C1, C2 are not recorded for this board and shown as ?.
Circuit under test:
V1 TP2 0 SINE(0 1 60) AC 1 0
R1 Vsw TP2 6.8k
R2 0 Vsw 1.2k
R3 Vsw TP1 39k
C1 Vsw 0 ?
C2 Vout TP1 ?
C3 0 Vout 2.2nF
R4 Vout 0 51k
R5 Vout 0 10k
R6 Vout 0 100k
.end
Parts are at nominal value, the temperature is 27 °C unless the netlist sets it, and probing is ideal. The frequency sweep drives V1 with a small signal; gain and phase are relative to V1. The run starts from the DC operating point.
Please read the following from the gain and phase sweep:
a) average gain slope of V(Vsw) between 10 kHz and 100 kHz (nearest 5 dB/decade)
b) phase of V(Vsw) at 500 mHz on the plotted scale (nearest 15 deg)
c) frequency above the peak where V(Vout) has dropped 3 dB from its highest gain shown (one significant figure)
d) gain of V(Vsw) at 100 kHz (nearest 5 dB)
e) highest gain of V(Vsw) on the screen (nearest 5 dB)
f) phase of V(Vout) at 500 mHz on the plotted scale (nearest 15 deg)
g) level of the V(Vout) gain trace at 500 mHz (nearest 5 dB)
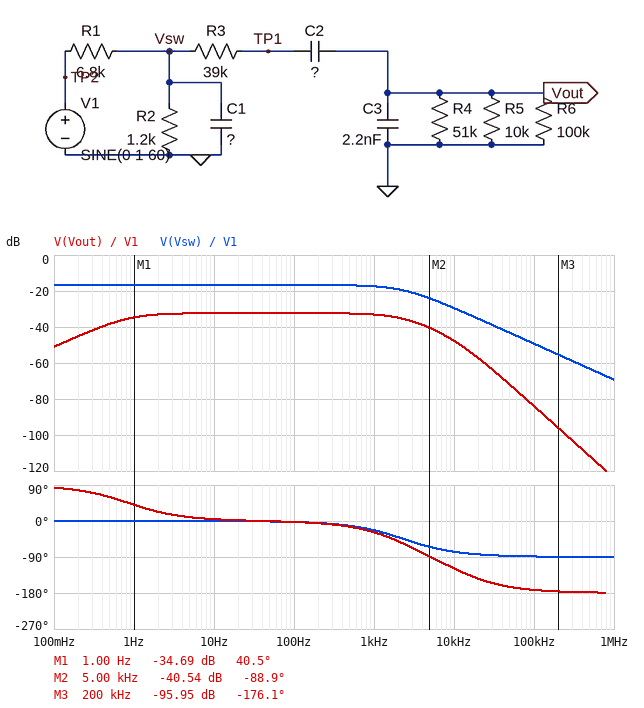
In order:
-20 dB/decade
0 deg
2 kHz
-50 dB
-15 dB
60 deg
-40 dB
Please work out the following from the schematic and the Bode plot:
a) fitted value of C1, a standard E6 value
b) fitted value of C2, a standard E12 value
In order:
68 nF
3.9 µF
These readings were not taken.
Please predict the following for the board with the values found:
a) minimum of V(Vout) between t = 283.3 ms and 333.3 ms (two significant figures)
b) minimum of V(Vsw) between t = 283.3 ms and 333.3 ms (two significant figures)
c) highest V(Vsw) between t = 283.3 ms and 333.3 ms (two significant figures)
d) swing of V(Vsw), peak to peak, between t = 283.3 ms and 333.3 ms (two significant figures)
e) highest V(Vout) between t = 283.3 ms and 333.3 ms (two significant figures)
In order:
-24 mV
-150 mV
150 mV
290 mV
24 mV
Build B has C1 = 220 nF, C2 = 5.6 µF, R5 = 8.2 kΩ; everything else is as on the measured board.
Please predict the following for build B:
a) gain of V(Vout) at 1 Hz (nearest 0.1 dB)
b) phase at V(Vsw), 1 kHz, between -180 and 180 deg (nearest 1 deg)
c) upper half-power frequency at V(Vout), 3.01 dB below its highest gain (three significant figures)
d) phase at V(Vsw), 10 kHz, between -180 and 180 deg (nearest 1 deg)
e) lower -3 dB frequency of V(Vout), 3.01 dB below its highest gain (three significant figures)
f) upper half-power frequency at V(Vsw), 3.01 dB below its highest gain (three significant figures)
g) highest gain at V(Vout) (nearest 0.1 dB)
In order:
-34.8 dB
-54 deg
724 Hz
-86 deg
609 mHz
693 Hz
-33.5 dB
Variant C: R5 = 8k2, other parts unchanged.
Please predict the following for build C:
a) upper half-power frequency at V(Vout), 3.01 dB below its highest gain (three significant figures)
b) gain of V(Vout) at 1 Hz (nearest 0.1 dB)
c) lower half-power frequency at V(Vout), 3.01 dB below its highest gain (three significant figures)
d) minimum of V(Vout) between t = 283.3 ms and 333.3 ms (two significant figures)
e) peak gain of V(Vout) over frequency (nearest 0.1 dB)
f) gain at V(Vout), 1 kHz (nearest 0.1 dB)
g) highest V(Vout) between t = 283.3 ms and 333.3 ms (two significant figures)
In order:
2.27 kHz
-35.9 dB
875 mHz
-21 mV
-33.5 dB
-34.2 dB
21 mV
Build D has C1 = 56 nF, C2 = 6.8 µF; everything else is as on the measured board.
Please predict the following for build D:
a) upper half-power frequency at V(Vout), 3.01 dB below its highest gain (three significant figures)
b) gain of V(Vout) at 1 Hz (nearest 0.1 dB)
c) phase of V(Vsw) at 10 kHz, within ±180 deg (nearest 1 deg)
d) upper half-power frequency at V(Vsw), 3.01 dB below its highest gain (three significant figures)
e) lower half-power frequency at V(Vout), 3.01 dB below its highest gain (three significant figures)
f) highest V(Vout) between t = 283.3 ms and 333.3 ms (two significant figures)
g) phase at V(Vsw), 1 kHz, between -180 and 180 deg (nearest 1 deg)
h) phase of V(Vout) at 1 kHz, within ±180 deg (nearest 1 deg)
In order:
2.69 kHz
-33.2 dB
-74 deg
2.72 kHz
490 mHz
24 mV
-19 deg
-24 deg
